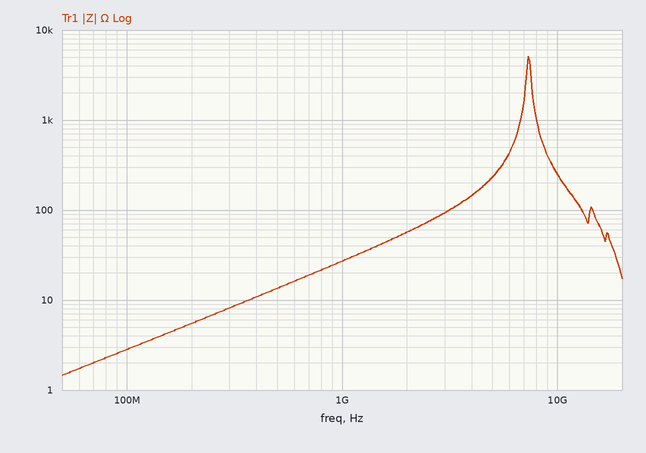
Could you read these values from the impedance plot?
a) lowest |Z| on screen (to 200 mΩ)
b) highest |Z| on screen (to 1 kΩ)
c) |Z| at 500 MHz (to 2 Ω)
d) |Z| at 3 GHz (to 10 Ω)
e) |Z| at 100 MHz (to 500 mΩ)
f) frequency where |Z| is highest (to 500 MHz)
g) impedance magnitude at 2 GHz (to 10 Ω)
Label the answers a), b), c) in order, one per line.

a) 1.4 Ω
b) 5 kΩ
c) 14 Ω
d) 90 Ω
e) 3.0 Ω
f) 7.5 GHz
g) 60 Ω
